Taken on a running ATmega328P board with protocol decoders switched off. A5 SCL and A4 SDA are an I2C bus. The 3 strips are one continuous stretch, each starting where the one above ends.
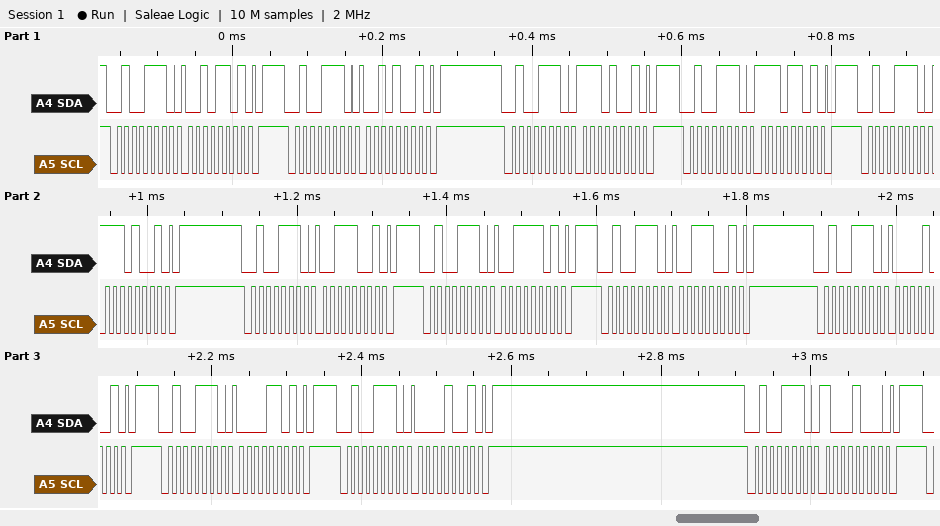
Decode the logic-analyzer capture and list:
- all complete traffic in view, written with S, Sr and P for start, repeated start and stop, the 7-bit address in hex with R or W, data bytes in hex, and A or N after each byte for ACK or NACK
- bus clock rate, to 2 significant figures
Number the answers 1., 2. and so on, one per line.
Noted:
1. S 27W A 2D A P S 27W A 29 A P S 27W A E9 A P S 27W A ED A P S 27W A E9 A P S 27W A 39 A P S 27W A 3D A P S 27W A 39 A P S 27W A 09 A P S 27W A 0D A P S 27W A 09 A P S 27W A 88 A P
2. 100 kHz
